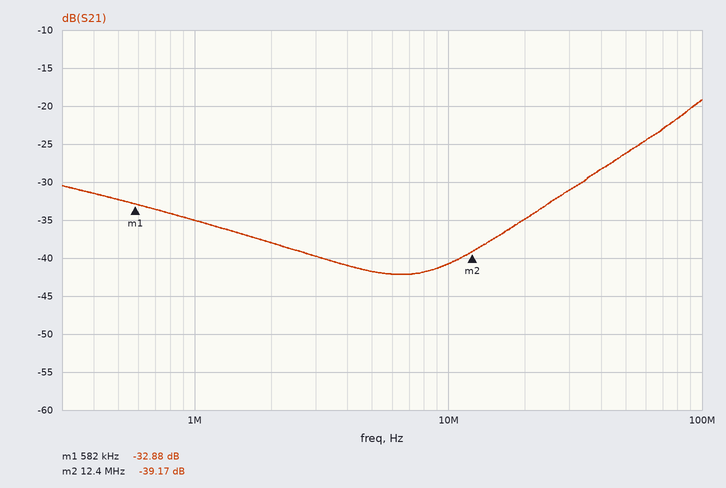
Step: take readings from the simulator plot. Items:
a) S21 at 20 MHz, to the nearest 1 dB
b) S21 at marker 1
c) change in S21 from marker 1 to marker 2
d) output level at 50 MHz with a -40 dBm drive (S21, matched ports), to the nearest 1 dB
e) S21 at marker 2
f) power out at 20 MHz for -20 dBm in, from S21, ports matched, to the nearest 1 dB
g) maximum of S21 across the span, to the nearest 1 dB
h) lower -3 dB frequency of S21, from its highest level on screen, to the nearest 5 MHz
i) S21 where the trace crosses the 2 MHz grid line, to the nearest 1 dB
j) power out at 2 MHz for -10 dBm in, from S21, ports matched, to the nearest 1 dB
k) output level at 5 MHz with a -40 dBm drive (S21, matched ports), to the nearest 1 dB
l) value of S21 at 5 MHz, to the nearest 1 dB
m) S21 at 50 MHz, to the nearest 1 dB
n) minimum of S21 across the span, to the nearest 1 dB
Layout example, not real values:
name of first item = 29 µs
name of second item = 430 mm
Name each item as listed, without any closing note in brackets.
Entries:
S21 at 20 MHz, to the nearest 1 dB = -35 dB
S21 at marker 1 = -32.88 dB
change in S21 from marker 1 to marker 2 = -6.29 dB
output level at 50 MHz with a -40 dBm drive (S21, matched ports), to the nearest 1 dB = -66 dBm
S21 at marker 2 = -39.17 dB
power out at 20 MHz for -20 dBm in, from S21, ports matched, to the nearest 1 dB = -55 dBm
maximum of S21 across the span, to the nearest 1 dB = -19 dB
lower -3 dB frequency of S21, from its highest level on screen, to the nearest 5 MHz = 75 MHz
S21 where the trace crosses the 2 MHz grid line, to the nearest 1 dB = -38 dB
power out at 2 MHz for -10 dBm in, from S21, ports matched, to the nearest 1 dB = -48 dBm
output level at 5 MHz with a -40 dBm drive (S21, matched ports), to the nearest 1 dB = -82 dBm
value of S21 at 5 MHz, to the nearest 1 dB = -42 dB
S21 at 50 MHz, to the nearest 1 dB = -26 dB
minimum of S21 across the span, to the nearest 1 dB = -42 dB
